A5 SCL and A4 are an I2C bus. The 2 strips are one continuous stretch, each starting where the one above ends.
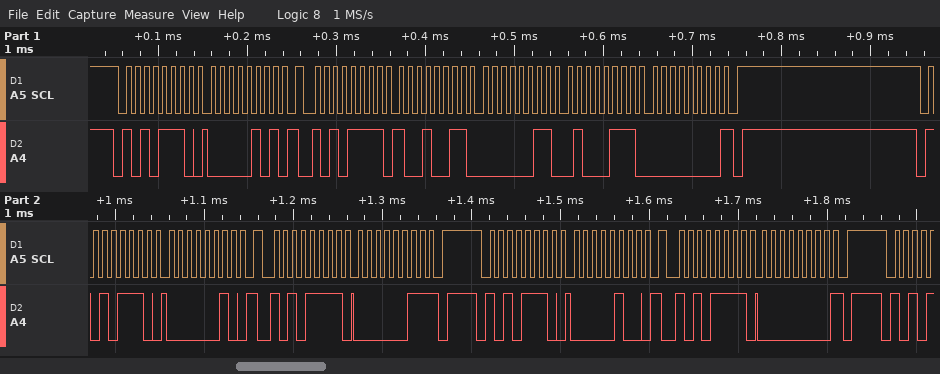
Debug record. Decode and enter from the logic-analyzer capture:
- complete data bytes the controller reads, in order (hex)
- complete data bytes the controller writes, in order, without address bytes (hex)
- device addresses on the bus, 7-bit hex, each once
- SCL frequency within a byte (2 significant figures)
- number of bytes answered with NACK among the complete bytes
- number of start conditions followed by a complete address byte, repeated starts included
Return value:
93 03 47 00 03 00
05 02 04
0x57
100 kHz
3
6
